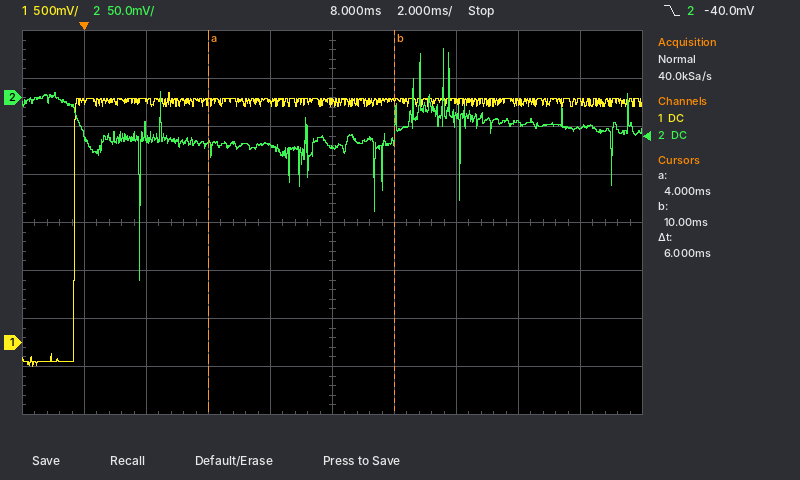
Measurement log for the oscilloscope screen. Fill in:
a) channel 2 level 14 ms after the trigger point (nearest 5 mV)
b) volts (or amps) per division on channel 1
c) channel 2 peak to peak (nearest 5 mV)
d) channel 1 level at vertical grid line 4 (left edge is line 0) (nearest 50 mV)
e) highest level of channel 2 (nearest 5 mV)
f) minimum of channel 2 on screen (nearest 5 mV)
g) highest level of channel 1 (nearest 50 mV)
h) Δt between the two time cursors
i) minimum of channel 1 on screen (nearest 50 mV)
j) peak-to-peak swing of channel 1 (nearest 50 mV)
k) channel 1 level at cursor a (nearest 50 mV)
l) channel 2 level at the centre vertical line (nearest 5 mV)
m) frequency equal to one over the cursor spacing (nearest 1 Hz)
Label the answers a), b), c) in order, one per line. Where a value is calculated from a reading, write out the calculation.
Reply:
a) -25 mV
b) 500 mV
c) 50 mV − (-190 mV) = 240 mV
d) 2.50 V
e) 50 mV
f) -190 mV
g) 2.60 V
h) 6 ms
i) -250 mV
j) 2.60 V − (-250 mV) = 2.85 V
k) 2.50 V
l) -50 mV
m) 1 / 6 ms ≈ 167 Hz
